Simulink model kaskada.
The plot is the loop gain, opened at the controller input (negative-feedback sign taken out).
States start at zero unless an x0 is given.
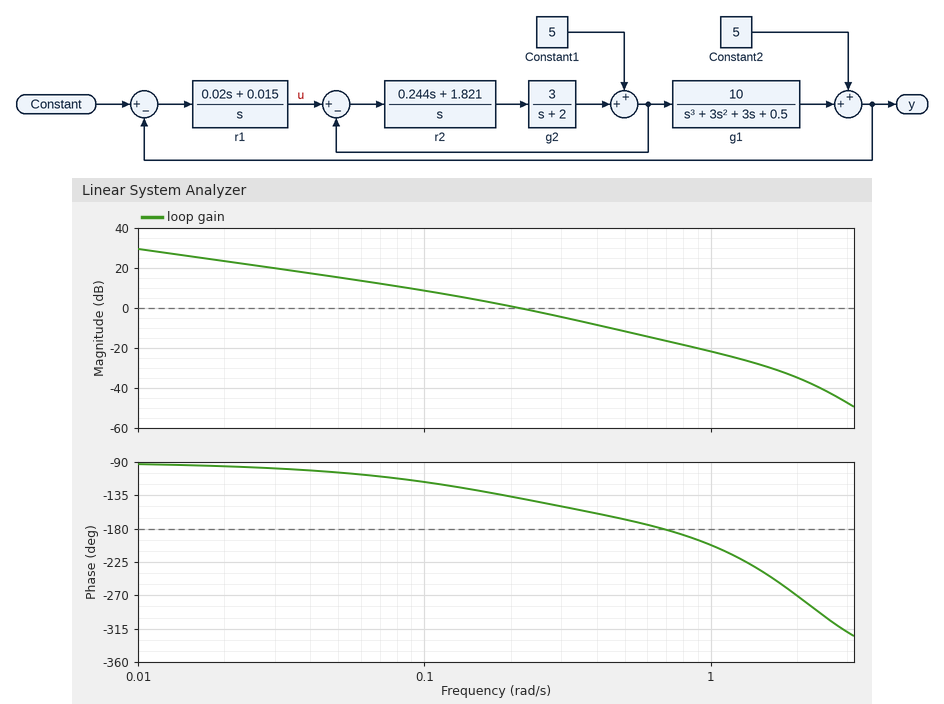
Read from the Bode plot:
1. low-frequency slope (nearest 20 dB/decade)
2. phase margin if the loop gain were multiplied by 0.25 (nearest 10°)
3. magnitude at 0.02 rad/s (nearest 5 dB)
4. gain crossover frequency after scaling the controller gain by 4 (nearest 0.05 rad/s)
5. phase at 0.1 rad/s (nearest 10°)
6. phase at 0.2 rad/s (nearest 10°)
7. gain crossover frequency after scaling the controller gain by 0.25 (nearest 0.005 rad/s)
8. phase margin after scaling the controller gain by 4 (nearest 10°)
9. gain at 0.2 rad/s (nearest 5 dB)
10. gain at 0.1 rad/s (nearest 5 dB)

-20 dB/decade
70°
25 dB
0.50 rad/s
-120°
-140°
0.070 rad/s
10°
0 dB
10 dB
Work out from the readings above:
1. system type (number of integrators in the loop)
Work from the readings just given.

1
